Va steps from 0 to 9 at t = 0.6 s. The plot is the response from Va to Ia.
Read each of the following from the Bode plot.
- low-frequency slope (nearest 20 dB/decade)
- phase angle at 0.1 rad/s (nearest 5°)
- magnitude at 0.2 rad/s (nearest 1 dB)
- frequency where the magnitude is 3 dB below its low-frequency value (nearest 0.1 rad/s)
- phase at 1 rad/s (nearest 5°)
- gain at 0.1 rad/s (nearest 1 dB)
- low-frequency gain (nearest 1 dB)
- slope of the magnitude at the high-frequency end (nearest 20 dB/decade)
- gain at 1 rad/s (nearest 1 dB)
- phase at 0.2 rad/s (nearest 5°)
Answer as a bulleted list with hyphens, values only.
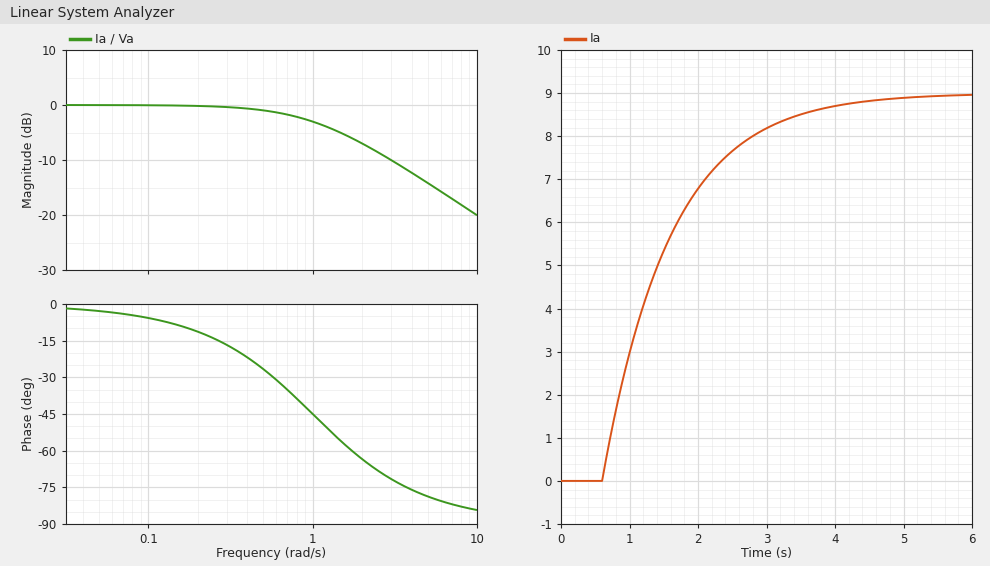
- 0 dB/decade
- -5°
- 0 dB
- 1.0 rad/s
- -45°
- 0 dB
- 0 dB
- -20 dB/decade
- -3 dB
- -10°
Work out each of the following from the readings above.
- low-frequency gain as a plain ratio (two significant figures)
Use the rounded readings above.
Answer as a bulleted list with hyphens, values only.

- 1.0
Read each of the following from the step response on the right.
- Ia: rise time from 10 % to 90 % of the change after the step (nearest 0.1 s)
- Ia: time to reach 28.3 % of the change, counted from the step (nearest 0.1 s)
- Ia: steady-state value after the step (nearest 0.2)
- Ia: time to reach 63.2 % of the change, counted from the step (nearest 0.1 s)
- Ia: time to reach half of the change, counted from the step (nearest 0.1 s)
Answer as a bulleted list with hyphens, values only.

- 2.2 s
- 0.3 s
- 9.0
- 1.0 s
- 0.7 s
